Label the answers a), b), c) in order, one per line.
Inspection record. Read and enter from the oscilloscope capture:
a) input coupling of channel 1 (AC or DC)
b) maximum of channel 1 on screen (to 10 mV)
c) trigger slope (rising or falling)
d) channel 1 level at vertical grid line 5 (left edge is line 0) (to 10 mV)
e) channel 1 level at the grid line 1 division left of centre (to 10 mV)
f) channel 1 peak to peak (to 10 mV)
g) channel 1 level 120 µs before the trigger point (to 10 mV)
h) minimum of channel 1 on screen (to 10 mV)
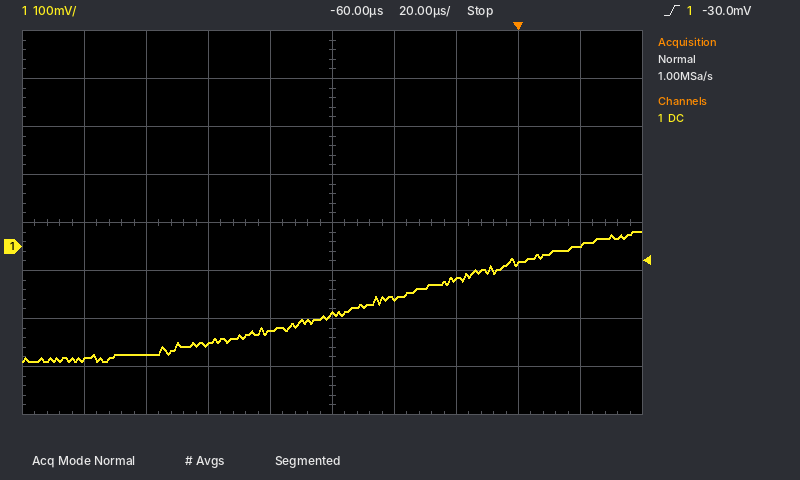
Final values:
a) DC
b) 30 mV
c) rising
d) -140 mV
e) -180 mV
f) 270 mV
g) -220 mV
h) -240 mV
